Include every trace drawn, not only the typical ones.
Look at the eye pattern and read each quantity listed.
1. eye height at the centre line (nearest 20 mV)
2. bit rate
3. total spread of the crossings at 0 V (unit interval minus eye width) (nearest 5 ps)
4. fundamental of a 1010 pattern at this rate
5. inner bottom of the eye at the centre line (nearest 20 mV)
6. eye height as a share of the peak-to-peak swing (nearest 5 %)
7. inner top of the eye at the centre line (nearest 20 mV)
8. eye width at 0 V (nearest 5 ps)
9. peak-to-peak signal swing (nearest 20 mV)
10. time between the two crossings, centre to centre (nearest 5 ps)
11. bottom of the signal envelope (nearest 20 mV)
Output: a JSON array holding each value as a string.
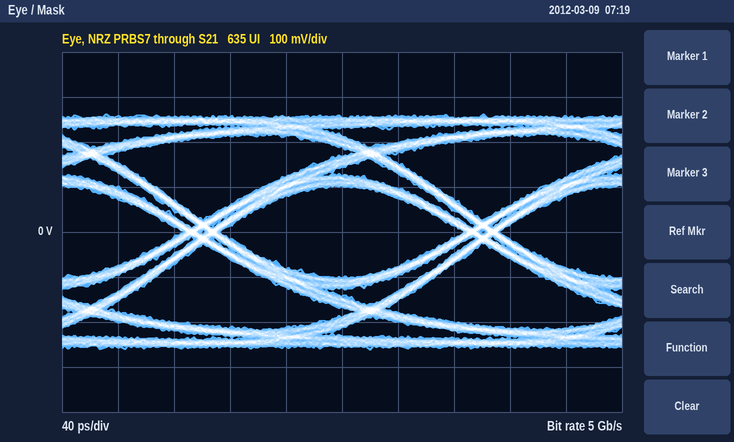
["200 mV", "5 Gb/s", "25 ps", "2.5 GHz", "-100 mV", "40 %", "100 mV", "175 ps", "520 mV", "200 ps", "-260 mV"]
